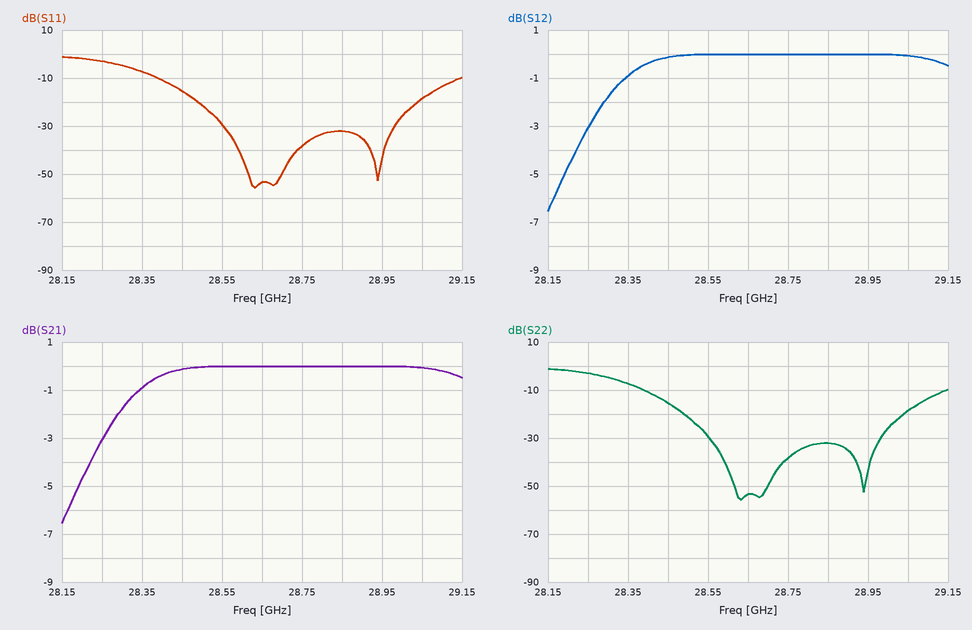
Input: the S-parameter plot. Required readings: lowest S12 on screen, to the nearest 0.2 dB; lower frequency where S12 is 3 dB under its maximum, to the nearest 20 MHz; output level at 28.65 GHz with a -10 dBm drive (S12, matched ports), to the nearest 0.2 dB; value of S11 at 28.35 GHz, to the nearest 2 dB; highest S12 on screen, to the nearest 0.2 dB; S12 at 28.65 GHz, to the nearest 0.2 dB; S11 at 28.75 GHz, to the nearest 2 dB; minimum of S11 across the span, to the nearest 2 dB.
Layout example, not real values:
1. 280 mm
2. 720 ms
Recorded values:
1. -6.6 dB
2. 28.26 GHz
3. -10.0 dBm
4. -8 dB
5. 0.0 dB
6. 0.0 dB
7. -38 dB
8. -56 dB
